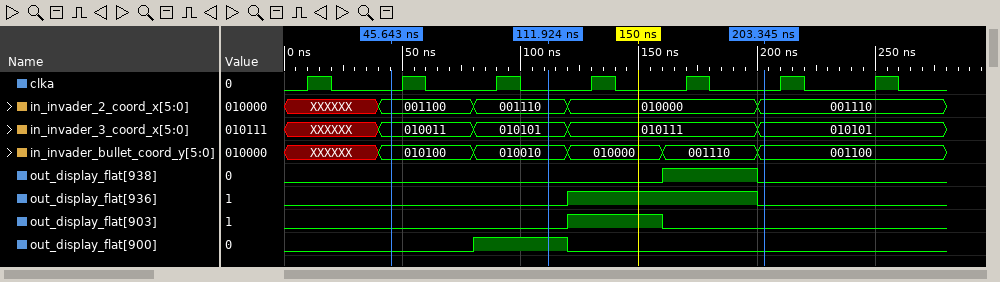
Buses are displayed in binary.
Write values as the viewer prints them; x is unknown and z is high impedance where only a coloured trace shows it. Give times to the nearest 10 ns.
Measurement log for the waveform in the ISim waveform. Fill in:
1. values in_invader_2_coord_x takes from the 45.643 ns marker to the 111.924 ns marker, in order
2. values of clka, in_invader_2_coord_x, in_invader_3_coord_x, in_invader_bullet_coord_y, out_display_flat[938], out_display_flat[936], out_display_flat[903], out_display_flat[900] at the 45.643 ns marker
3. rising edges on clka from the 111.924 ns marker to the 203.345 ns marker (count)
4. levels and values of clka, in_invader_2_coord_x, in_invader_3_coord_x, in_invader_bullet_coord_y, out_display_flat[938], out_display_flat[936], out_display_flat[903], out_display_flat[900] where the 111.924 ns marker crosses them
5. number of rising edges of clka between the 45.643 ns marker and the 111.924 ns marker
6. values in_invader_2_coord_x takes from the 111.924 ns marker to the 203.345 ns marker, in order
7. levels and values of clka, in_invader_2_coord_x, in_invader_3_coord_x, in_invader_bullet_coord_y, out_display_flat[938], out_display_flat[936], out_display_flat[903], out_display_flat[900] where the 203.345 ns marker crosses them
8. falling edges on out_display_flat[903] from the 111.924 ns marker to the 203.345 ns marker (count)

001100, 001110
clka=0, in_invader_2_coord_x=001100, in_invader_3_coord_x=010011, in_invader_bullet_coord_y=010100, out_display_flat[938]=0, out_display_flat[936]=0, out_display_flat[903]=0, out_display_flat[900]=0
2
clka=0, in_invader_2_coord_x=001110, in_invader_3_coord_x=010101, in_invader_bullet_coord_y=010010, out_display_flat[938]=0, out_display_flat[936]=0, out_display_flat[903]=0, out_display_flat[900]=1
2
001110, 010000, 001110
clka=0, in_invader_2_coord_x=001110, in_invader_3_coord_x=010101, in_invader_bullet_coord_y=001100, out_display_flat[938]=0, out_display_flat[936]=0, out_display_flat[903]=0, out_display_flat[900]=0
1
